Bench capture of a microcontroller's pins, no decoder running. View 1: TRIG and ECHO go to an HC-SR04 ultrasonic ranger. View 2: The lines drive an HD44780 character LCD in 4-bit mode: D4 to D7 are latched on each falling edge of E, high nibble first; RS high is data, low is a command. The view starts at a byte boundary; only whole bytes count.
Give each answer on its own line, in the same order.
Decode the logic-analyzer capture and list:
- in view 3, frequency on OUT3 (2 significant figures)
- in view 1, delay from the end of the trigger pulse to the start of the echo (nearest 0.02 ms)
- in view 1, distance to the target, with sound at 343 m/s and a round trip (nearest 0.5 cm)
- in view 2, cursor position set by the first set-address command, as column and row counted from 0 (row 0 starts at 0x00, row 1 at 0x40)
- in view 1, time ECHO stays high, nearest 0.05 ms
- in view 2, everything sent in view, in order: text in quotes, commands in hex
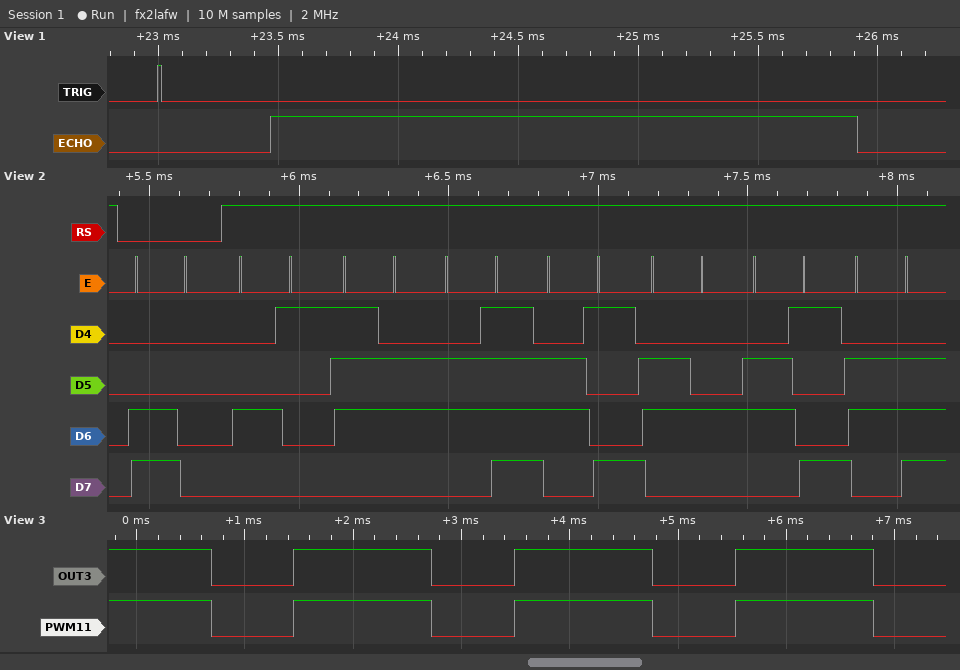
490 Hz
0.46 ms
42 cm
column 0, row 1
2.45 ms
0xC0 "Avoidin"
